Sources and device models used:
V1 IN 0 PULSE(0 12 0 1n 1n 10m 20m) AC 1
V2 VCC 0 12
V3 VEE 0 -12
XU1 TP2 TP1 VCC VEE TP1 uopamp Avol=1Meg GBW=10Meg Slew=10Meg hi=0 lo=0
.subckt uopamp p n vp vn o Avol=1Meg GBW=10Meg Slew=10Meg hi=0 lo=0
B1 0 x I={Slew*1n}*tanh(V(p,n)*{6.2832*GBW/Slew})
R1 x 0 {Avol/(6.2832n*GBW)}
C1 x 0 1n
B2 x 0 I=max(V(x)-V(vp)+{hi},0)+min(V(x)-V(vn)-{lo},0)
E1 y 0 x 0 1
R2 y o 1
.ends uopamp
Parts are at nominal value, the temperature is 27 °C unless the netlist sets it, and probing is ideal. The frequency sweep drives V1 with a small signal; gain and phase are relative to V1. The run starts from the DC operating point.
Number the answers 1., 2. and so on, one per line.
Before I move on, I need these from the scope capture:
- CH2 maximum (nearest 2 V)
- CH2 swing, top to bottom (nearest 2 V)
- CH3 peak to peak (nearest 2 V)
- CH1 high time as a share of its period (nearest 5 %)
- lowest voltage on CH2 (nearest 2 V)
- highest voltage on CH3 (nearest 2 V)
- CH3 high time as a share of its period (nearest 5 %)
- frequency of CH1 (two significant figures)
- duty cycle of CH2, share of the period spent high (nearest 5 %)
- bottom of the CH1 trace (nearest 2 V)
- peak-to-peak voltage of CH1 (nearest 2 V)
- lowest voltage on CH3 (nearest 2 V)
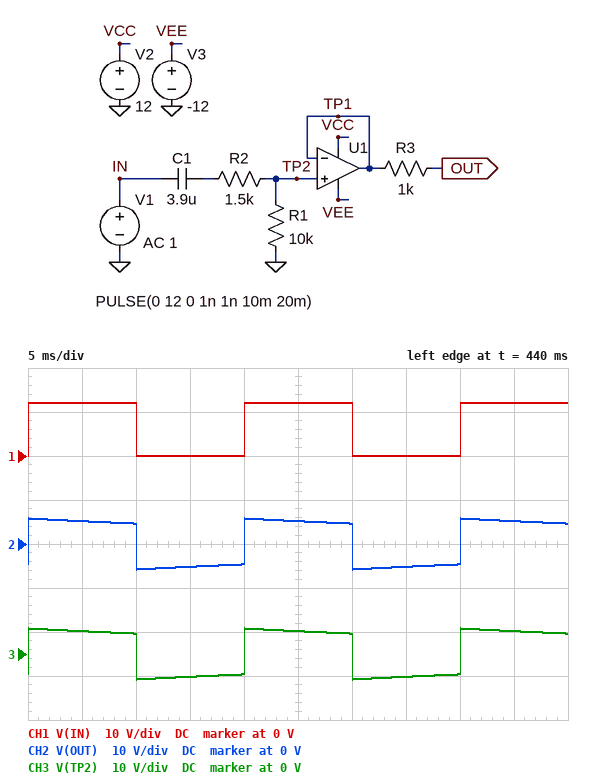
1. 6 V
2. 12 V
3. 12 V
4. 50 %
5. -6 V
6. 6 V
7. 50 %
8. 50 Hz
9. 50 %
10. 0 V
11. 12 V
12. -6 V
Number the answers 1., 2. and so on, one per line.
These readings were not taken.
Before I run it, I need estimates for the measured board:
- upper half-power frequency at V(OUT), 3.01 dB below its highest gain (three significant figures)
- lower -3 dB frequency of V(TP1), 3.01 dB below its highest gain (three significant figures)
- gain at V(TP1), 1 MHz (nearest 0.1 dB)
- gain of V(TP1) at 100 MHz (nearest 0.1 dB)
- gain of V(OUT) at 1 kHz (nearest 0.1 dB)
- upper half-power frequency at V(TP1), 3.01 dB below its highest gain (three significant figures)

1. 10.0 MHz
2. 3.55 Hz
3. -1.3 dB
4. -21.3 dB
5. -1.2 dB
6. 10.0 MHz
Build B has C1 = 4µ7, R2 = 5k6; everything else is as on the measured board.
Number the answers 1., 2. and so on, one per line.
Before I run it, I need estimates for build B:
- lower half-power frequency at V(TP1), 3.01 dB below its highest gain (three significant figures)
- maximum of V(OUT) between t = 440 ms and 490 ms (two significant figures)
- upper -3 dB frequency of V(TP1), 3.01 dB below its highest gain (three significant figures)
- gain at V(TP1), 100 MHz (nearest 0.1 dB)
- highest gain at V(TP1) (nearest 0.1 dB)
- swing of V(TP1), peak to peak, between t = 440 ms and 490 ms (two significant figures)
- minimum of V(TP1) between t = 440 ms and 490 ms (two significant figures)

1. 2.17 Hz
2. 4.1 V
3. 10.0 MHz
4. -23.9 dB
5. -3.9 dB
6. 8.2 V
7. -4.1 V
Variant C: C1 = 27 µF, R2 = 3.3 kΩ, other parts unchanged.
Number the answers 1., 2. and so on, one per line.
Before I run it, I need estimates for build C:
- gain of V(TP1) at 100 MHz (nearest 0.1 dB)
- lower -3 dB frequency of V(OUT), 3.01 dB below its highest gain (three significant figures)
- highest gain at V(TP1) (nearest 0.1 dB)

1. -22.5 dB
2. 443 mHz
3. -2.5 dB
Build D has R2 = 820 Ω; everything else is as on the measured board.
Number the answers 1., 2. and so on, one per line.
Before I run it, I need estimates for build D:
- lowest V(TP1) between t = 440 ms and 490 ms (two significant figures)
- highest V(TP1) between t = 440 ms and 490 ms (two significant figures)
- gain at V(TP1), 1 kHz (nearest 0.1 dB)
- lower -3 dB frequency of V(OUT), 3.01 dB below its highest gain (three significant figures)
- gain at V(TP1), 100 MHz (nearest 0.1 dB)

1. -6.2 V
2. 6.2 V
3. -0.7 dB
4. 3.77 Hz
5. -20.7 dB
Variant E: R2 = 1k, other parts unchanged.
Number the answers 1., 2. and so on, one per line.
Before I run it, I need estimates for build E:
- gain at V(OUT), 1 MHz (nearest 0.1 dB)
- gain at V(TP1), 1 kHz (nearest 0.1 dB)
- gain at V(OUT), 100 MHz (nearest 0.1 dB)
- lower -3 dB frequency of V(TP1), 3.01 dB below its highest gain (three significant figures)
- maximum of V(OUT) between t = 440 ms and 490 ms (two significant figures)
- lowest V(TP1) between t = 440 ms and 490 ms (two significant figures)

1. -0.9 dB
2. -0.8 dB
3. -20.9 dB
4. 3.71 Hz
5. 6.1 V
6. -6.1 V
